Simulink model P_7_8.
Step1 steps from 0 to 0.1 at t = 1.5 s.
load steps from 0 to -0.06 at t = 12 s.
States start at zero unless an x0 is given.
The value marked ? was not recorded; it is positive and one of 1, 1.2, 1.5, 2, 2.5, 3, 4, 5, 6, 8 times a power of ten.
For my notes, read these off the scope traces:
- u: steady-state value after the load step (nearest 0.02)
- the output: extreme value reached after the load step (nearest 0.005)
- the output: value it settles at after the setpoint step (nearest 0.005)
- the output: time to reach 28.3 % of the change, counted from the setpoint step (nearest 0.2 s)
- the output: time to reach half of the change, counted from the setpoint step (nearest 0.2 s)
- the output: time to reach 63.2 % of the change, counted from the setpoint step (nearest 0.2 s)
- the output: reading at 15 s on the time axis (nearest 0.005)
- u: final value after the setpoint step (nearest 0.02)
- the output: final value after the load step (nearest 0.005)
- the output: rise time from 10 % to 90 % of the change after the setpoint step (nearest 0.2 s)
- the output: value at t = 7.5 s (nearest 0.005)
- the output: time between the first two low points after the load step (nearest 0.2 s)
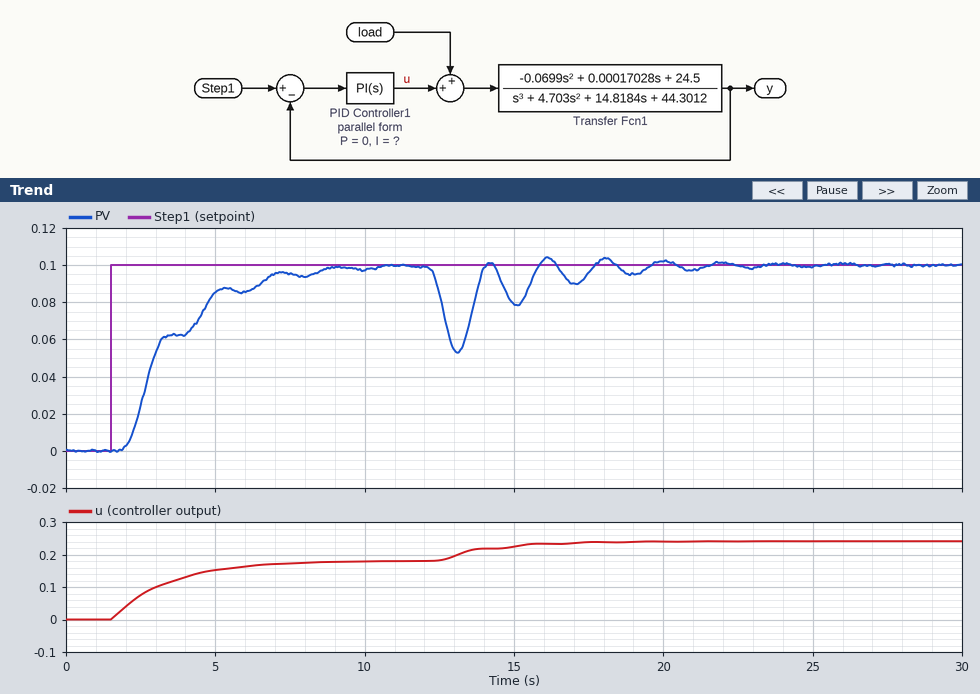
0.24
0.055
0.100
1.0 s
1.4 s
2.6 s
0.080
0.18
0.100
4.2 s
0.095
2.0 s
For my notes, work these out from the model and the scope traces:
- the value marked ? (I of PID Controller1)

0.8
